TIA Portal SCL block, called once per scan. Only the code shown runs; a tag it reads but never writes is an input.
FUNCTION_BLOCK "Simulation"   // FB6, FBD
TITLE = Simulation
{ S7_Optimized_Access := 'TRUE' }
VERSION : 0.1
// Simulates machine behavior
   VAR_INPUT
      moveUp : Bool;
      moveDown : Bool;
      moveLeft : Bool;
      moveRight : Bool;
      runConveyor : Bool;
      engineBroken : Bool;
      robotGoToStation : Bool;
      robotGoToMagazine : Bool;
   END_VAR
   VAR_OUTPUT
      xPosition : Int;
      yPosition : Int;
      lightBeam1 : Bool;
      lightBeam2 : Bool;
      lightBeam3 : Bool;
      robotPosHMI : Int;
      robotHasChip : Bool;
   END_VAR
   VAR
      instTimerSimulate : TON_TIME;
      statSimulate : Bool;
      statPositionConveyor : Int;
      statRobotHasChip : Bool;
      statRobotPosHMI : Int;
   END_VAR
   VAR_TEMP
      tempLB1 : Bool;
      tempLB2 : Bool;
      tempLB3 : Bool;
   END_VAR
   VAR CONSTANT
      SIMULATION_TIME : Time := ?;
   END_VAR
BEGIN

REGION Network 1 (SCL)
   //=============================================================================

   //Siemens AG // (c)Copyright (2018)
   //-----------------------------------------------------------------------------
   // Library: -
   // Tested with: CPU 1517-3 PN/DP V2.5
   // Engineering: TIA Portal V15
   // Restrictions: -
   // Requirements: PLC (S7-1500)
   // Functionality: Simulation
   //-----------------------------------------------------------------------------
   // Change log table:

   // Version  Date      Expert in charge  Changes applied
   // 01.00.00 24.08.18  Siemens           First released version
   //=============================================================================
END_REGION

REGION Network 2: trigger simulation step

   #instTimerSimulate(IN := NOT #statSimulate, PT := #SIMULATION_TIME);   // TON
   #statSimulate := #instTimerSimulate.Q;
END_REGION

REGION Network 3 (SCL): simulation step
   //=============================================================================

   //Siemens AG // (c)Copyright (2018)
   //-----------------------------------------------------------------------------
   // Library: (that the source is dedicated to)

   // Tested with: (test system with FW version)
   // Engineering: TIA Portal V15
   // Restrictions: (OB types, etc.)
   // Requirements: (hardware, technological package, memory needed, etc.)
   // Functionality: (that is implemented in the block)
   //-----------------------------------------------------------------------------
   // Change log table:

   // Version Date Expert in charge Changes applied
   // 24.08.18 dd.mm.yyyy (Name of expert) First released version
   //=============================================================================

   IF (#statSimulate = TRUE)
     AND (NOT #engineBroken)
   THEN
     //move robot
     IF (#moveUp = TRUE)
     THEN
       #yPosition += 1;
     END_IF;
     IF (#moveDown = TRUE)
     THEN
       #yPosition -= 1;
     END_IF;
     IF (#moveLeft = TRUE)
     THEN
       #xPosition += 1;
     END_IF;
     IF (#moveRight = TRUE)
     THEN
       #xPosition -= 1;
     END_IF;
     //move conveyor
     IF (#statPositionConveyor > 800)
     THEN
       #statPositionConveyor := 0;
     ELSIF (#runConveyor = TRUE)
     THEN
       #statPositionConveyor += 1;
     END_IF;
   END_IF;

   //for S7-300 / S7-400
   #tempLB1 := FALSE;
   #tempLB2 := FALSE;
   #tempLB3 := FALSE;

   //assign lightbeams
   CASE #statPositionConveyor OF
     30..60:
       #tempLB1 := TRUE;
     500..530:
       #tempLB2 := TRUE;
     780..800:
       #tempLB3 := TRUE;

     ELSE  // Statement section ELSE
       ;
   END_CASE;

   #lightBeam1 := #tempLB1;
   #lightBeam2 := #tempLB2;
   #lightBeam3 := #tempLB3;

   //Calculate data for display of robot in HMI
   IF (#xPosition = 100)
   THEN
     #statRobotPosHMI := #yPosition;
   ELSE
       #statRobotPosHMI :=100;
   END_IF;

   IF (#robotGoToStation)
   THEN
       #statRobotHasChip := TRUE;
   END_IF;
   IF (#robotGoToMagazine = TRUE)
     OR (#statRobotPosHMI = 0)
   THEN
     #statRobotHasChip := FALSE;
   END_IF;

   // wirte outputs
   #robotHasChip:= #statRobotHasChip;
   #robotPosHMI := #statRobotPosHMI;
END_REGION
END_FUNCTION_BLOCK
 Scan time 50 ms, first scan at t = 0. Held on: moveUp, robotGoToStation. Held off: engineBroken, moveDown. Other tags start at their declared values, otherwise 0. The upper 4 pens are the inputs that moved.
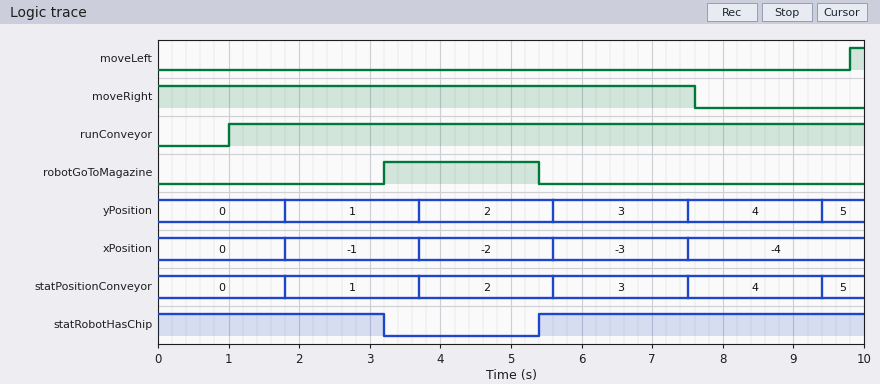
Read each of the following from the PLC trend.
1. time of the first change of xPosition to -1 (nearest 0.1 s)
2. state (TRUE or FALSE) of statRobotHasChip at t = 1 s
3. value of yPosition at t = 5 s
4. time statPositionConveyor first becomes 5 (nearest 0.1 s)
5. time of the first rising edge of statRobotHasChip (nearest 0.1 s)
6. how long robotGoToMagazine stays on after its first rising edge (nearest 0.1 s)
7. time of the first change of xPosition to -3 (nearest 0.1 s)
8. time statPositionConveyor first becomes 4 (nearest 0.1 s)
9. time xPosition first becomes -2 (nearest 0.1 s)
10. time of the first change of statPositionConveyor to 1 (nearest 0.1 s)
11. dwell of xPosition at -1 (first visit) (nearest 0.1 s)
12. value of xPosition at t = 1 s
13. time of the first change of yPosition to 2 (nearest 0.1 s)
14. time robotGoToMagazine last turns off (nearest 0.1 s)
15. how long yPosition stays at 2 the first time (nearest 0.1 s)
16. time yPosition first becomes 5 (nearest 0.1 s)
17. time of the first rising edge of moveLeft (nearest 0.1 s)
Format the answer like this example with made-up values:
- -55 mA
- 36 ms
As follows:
- 1.8 s
- TRUE
- 2
- 9.4 s
- 5.4 s
- 2.2 s
- 5.6 s
- 7.5 s
- 3.7 s
- 1.8 s
- 1.9 s
- 0
- 3.7 s
- 5.4 s
- 1.9 s
- 9.4 s
- 9.8 s
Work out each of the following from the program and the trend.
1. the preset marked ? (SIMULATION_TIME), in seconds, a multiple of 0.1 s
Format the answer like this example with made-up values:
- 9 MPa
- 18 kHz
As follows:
- 1.8 s
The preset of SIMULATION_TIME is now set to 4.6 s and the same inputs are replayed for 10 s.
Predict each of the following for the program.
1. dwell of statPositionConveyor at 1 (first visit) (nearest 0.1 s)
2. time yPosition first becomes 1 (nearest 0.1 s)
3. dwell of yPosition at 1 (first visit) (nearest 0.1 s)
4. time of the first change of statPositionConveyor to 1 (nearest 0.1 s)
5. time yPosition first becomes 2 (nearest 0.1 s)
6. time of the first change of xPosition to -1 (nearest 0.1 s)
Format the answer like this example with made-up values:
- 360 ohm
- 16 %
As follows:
- 4.7 s
- 4.6 s
- 4.7 s
- 4.6 s
- 9.3 s
- 4.6 s
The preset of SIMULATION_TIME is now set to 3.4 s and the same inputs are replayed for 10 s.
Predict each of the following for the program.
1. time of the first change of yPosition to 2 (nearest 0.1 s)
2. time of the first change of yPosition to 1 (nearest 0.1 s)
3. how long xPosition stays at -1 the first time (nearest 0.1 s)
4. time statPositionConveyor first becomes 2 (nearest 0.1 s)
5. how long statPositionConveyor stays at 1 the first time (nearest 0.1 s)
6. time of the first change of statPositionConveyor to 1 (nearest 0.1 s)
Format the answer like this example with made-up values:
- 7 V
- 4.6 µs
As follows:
- 6.9 s
- 3.4 s
- 3.5 s
- 6.9 s
- 3.5 s
- 3.4 s
